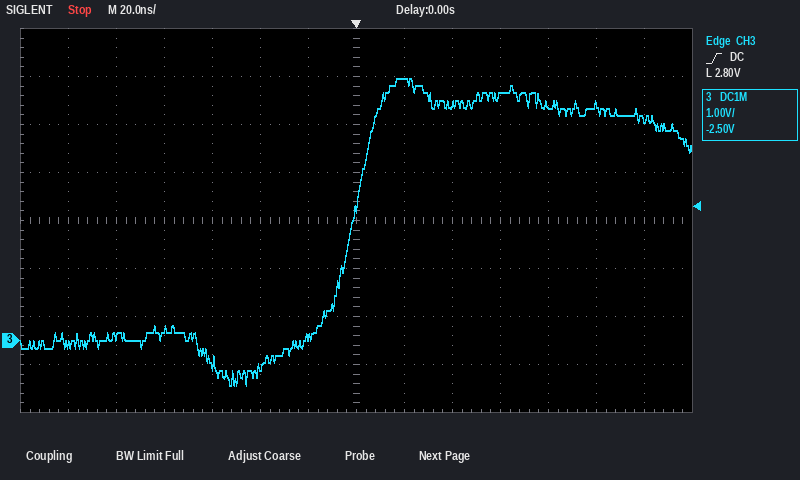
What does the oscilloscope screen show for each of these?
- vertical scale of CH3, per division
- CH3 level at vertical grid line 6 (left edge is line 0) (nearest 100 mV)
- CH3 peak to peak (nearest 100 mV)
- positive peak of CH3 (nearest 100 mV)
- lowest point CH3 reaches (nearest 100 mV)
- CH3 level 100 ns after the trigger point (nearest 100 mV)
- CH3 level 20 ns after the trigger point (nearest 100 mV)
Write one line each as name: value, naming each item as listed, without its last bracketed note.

vertical scale of CH3, per division: 1 V
CH3 level at vertical grid line 6 (left edge is line 0): 100 mV
CH3 peak to peak: 6.4 V
positive peak of CH3: 5.5 V
lowest point CH3 reaches: -900 mV
CH3 level 100 ns after the trigger point: 4.9 V
CH3 level 20 ns after the trigger point: 5.5 V
